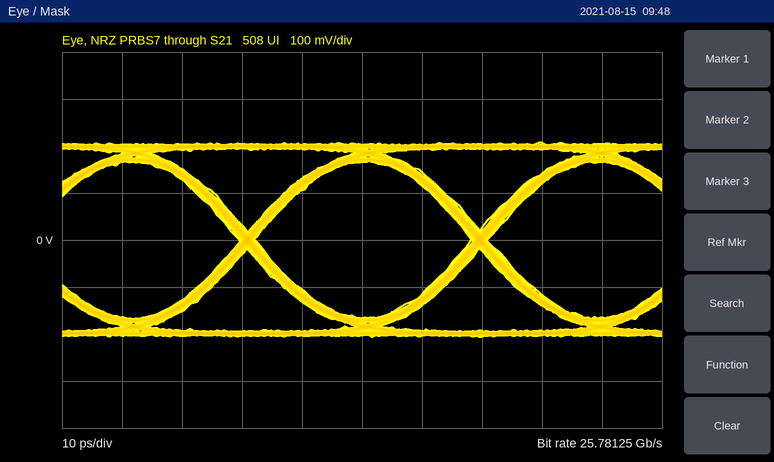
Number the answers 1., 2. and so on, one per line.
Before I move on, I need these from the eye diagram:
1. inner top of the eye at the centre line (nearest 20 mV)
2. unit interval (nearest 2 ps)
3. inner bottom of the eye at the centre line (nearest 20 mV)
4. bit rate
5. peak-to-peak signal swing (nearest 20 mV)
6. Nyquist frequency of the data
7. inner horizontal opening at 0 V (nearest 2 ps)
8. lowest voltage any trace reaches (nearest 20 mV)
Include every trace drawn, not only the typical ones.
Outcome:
1. 160 mV
2. 38 ps
3. -160 mV
4. 25.78125 Gb/s
5. 420 mV
6. 12.89062 GHz
7. 36 ps
8. -200 mV
